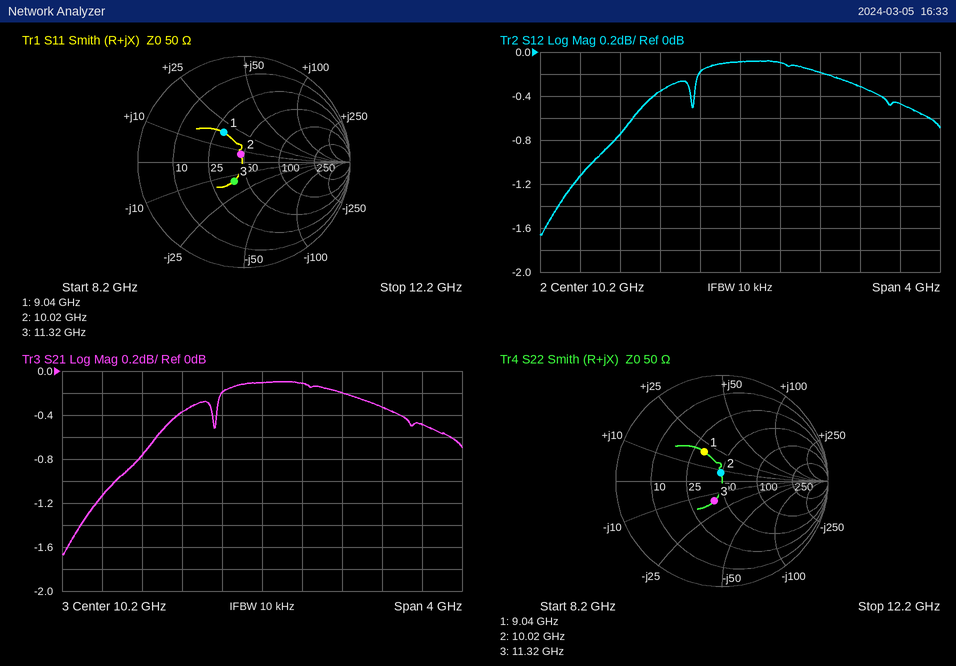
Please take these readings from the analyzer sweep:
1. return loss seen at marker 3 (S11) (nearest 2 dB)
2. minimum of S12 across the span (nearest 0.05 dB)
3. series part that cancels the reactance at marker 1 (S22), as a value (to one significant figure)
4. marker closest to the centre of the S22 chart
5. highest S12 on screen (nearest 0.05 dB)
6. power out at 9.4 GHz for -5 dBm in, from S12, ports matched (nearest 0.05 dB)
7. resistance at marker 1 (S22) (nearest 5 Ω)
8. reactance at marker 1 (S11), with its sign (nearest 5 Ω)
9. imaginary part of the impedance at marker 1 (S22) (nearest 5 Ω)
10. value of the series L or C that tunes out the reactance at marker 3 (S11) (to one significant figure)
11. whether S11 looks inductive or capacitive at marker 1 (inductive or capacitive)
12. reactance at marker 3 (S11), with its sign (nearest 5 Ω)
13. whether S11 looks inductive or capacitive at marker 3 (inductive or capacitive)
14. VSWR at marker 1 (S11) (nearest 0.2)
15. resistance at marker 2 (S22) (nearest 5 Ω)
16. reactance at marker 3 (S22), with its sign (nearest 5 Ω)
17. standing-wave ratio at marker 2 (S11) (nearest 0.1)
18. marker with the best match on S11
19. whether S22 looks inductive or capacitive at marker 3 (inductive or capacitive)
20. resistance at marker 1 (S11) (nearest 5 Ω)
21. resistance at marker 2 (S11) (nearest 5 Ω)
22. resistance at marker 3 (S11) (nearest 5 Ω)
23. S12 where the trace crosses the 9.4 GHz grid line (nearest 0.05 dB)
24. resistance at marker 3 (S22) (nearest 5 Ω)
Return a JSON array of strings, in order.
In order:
["14 dB", "-1.65 dB", "900 fF", "marker 2", "-0.10 dB", "-5.35 dBm", "30 Ω", "+20 Ω", "+20 Ω", "200 pH", "inductive", "-15 Ω", "capacitive", "2.0", "50 Ω", "-15 Ω", "1.2", "marker 2", "capacitive", "30 Ω", "45 Ω", "40 Ω", "-0.35 dB", "40 Ω"]
